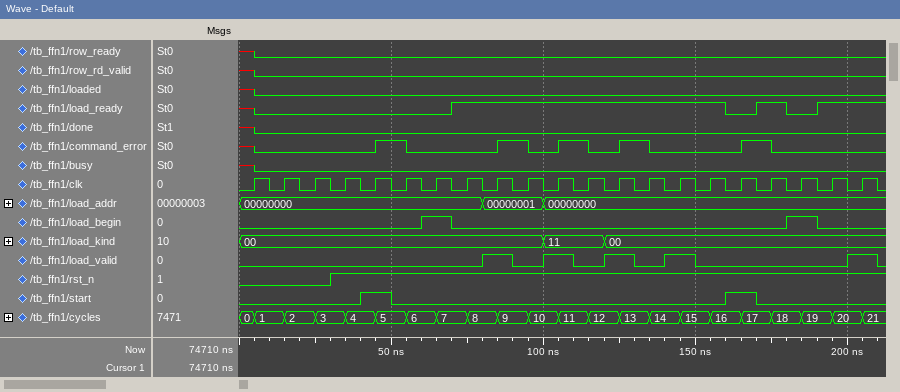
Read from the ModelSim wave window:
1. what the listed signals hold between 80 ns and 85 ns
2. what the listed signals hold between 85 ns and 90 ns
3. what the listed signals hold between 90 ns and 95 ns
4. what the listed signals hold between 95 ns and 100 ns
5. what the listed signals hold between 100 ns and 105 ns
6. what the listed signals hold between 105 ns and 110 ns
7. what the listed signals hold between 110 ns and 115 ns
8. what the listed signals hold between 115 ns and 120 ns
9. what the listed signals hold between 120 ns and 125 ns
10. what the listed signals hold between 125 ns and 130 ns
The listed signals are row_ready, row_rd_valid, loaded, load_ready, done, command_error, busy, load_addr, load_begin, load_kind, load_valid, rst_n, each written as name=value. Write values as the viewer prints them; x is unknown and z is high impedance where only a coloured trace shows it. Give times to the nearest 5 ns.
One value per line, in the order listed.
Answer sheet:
row_ready=0, row_rd_valid=0, loaded=0, load_ready=1, done=0, command_error=0, busy=0, load_addr=00000001, load_begin=0, load_kind=00, load_valid=1, rst_n=1
row_ready=0, row_rd_valid=0, loaded=0, load_ready=1, done=0, command_error=1, busy=0, load_addr=00000001, load_begin=0, load_kind=00, load_valid=1, rst_n=1
row_ready=0, row_rd_valid=0, loaded=0, load_ready=1, done=0, command_error=1, busy=0, load_addr=00000001, load_begin=0, load_kind=00, load_valid=0, rst_n=1
row_ready=0, row_rd_valid=0, loaded=0, load_ready=1, done=0, command_error=0, busy=0, load_addr=00000001, load_begin=0, load_kind=00, load_valid=0, rst_n=1
row_ready=0, row_rd_valid=0, loaded=0, load_ready=1, done=0, command_error=0, busy=0, load_addr=00000000, load_begin=0, load_kind=11, load_valid=1, rst_n=1
row_ready=0, row_rd_valid=0, loaded=0, load_ready=1, done=0, command_error=1, busy=0, load_addr=00000000, load_begin=0, load_kind=11, load_valid=1, rst_n=1
row_ready=0, row_rd_valid=0, loaded=0, load_ready=1, done=0, command_error=1, busy=0, load_addr=00000000, load_begin=0, load_kind=11, load_valid=0, rst_n=1
row_ready=0, row_rd_valid=0, loaded=0, load_ready=1, done=0, command_error=0, busy=0, load_addr=00000000, load_begin=0, load_kind=11, load_valid=0, rst_n=1
row_ready=0, row_rd_valid=0, loaded=0, load_ready=1, done=0, command_error=0, busy=0, load_addr=00000000, load_begin=0, load_kind=00, load_valid=1, rst_n=1
row_ready=0, row_rd_valid=0, loaded=0, load_ready=1, done=0, command_error=1, busy=0, load_addr=00000000, load_begin=0, load_kind=00, load_valid=1, rst_n=1
